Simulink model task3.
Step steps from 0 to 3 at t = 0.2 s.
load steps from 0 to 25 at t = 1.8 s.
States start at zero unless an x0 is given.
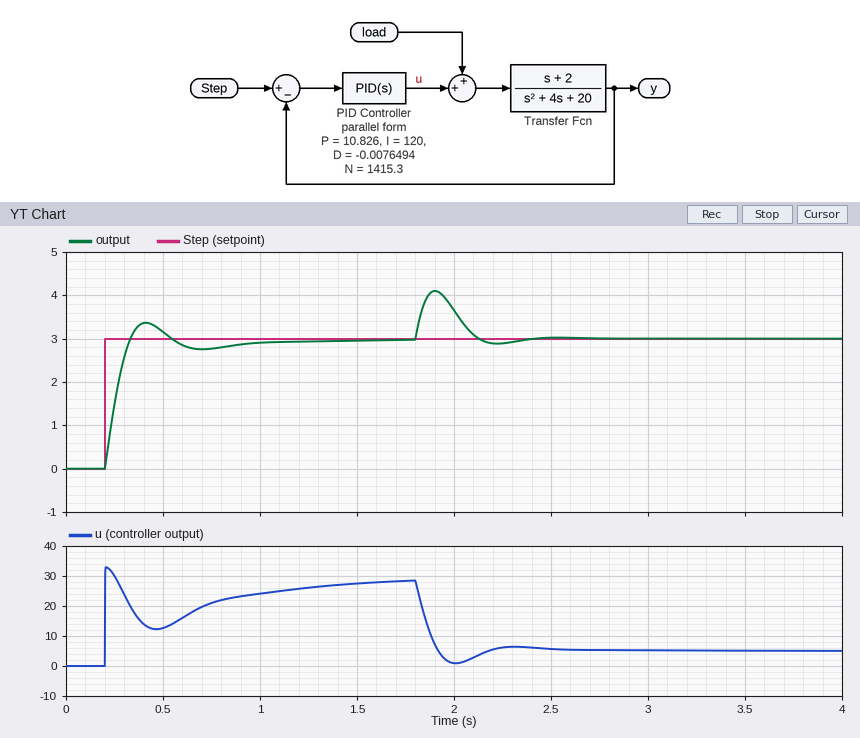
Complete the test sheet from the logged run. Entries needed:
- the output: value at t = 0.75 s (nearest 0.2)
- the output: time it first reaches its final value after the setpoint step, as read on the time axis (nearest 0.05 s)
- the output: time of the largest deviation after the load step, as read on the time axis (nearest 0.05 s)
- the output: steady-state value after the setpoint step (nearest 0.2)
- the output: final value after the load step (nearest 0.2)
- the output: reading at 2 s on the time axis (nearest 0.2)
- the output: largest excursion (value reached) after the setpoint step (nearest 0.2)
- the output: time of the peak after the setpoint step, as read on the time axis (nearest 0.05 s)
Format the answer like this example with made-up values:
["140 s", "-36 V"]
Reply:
["2.8", "0.35 s", "1.90 s", "3.0", "3.0", "3.6", "3.4", "0.40 s"]
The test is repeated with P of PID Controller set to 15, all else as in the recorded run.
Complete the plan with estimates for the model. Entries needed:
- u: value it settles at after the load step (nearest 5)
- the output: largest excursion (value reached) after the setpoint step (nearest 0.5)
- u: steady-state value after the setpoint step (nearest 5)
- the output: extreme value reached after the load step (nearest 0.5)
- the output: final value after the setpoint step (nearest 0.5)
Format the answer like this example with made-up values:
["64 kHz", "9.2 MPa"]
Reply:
["5", "3.0", "30", "4.0", "3.0"]
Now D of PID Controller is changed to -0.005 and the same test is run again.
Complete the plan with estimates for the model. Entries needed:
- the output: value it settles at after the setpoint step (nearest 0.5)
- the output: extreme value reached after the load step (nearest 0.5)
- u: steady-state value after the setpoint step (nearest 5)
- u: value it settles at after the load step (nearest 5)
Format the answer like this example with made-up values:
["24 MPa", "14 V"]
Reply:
["3.0", "4.0", "30", "5"]
